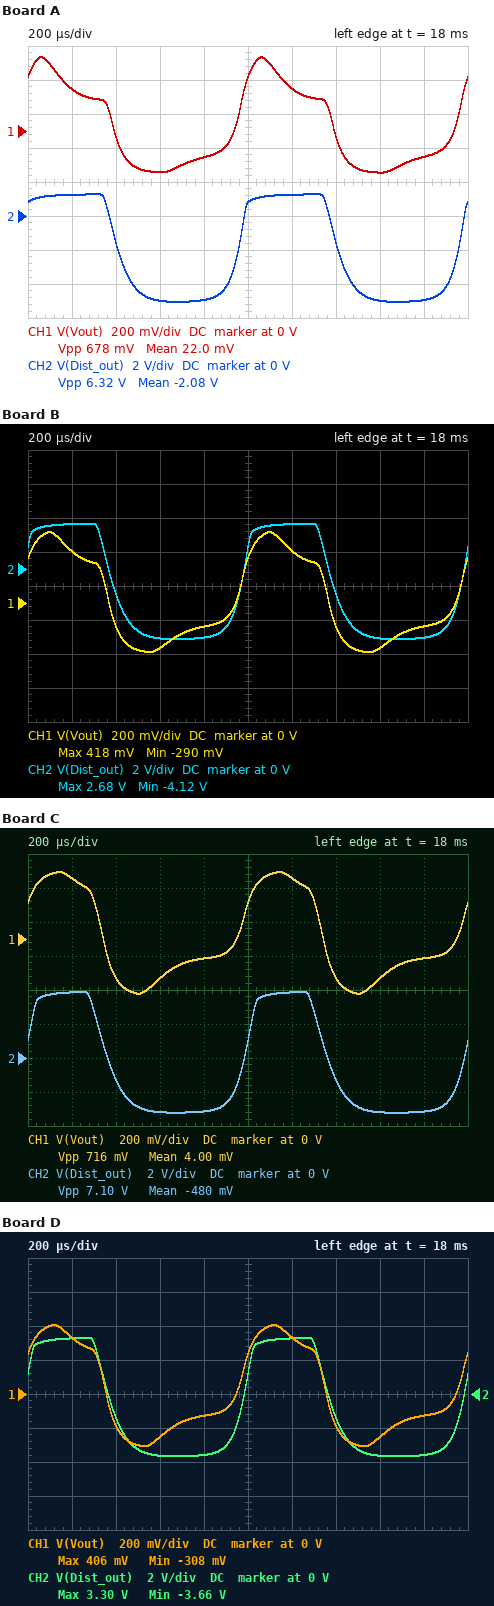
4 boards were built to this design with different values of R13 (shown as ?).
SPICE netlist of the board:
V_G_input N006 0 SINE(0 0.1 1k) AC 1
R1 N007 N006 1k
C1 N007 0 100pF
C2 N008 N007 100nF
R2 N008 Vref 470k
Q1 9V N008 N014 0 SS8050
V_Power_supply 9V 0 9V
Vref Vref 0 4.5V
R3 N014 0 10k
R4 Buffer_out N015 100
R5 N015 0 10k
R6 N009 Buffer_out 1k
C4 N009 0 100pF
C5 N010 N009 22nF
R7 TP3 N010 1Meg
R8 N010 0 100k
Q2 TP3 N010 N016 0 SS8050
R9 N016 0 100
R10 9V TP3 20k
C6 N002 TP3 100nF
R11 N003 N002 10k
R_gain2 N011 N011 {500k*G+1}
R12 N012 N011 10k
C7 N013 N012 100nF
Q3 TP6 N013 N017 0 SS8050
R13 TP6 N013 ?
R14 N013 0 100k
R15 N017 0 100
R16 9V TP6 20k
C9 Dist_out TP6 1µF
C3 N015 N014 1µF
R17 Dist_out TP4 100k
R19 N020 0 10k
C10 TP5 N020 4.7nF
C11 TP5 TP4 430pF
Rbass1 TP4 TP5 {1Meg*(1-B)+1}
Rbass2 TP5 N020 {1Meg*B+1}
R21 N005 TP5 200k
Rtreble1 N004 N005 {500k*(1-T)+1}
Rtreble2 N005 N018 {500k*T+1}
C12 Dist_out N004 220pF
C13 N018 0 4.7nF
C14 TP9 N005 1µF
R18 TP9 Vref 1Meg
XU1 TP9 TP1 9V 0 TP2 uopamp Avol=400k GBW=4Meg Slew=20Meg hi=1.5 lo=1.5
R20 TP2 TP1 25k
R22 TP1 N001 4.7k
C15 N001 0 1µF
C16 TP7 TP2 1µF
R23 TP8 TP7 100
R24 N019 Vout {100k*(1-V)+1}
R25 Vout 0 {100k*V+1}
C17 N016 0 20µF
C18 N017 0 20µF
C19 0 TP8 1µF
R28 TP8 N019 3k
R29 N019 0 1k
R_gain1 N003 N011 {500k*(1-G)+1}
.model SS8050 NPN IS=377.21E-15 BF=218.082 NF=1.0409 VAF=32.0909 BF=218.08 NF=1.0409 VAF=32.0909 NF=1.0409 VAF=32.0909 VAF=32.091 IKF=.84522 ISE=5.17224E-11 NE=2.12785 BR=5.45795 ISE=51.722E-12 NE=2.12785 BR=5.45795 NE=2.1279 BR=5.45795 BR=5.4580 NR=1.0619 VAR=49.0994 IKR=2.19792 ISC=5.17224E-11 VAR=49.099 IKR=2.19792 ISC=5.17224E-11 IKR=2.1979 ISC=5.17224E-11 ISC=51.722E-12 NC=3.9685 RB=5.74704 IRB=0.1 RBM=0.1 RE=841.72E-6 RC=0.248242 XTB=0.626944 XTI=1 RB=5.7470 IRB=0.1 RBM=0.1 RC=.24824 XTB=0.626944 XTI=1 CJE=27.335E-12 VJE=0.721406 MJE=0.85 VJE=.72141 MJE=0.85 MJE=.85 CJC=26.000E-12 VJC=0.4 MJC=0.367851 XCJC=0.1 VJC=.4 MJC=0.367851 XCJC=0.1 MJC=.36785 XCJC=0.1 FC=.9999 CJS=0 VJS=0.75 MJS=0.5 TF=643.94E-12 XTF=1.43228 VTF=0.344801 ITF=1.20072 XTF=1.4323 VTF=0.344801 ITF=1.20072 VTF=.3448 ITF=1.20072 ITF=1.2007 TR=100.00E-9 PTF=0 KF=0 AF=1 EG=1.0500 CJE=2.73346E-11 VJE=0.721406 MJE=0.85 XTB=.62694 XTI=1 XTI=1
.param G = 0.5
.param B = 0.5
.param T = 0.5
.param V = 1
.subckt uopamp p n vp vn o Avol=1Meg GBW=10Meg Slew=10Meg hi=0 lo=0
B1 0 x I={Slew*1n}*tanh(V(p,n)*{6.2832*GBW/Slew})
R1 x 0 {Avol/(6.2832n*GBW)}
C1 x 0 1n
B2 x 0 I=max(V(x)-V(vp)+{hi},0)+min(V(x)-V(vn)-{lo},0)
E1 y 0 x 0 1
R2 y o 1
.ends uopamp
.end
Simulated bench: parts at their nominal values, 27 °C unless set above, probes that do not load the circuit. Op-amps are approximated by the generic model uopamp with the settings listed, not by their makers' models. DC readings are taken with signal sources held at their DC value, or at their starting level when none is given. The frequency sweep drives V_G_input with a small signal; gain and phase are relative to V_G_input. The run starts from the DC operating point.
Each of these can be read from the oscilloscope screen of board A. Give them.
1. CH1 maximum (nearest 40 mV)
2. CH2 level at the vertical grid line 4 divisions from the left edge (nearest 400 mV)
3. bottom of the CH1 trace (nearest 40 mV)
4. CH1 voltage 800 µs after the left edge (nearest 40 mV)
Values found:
440 mV
-4.8 V
-240 mV
-160 mV
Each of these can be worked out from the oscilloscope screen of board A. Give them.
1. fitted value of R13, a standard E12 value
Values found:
1.2 MΩ
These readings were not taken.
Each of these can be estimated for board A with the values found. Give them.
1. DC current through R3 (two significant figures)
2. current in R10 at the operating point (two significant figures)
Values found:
290 µA
110 µA
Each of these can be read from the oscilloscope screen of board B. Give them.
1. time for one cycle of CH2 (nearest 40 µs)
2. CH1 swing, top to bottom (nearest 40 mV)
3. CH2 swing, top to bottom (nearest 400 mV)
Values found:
1.00 ms
720 mV
6.8 V
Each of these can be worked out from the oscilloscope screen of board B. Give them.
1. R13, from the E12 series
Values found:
820 kΩ
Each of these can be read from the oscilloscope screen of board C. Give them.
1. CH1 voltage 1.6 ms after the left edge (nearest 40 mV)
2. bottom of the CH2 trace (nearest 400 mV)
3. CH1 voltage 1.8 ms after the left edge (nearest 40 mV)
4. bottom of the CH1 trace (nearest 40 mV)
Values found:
-240 mV
-3.2 V
-120 mV
-320 mV
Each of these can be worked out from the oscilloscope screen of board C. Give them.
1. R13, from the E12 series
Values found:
560 kΩ
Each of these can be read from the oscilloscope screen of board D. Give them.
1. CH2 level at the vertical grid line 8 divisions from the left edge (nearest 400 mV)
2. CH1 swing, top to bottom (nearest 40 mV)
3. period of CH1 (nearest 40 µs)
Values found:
-3.6 V
720 mV
1.00 ms
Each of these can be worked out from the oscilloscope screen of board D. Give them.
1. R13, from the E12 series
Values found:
680 kΩ
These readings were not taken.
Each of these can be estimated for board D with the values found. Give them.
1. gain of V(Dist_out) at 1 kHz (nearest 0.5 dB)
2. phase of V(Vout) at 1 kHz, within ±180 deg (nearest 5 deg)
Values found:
38.5 dB
60 deg
